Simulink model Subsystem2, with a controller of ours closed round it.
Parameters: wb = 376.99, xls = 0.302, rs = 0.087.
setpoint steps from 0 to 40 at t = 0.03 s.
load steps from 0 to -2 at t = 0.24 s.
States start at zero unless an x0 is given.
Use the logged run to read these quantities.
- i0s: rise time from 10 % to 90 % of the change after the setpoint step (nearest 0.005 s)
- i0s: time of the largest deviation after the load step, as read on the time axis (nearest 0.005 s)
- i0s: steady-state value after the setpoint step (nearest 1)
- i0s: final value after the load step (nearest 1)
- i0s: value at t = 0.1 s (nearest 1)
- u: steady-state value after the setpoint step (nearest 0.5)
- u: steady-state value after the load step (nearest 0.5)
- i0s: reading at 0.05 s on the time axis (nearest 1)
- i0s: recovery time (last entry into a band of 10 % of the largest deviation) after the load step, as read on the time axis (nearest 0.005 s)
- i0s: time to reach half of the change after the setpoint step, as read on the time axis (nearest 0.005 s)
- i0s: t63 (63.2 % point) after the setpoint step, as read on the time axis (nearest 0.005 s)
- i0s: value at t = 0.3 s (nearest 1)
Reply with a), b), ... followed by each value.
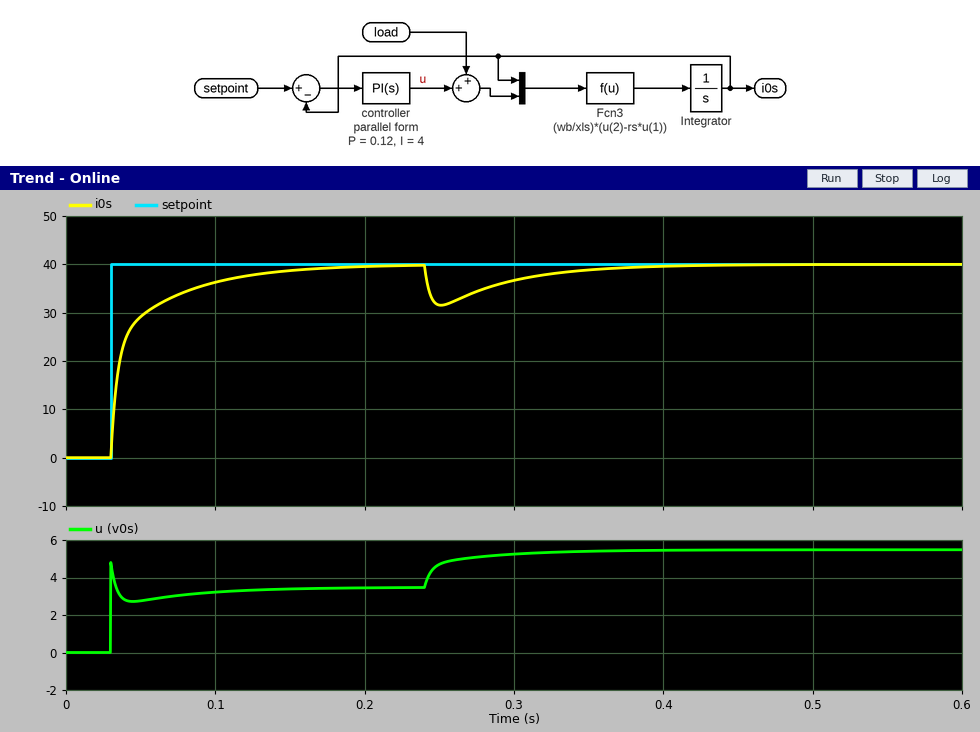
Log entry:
a) 0.065 s
b) 0.250 s
c) 40
d) 40
e) 36
f) 3.5
g) 5.5
h) 29
i) 0.365 s
j) 0.035 s
k) 0.040 s
l) 37
